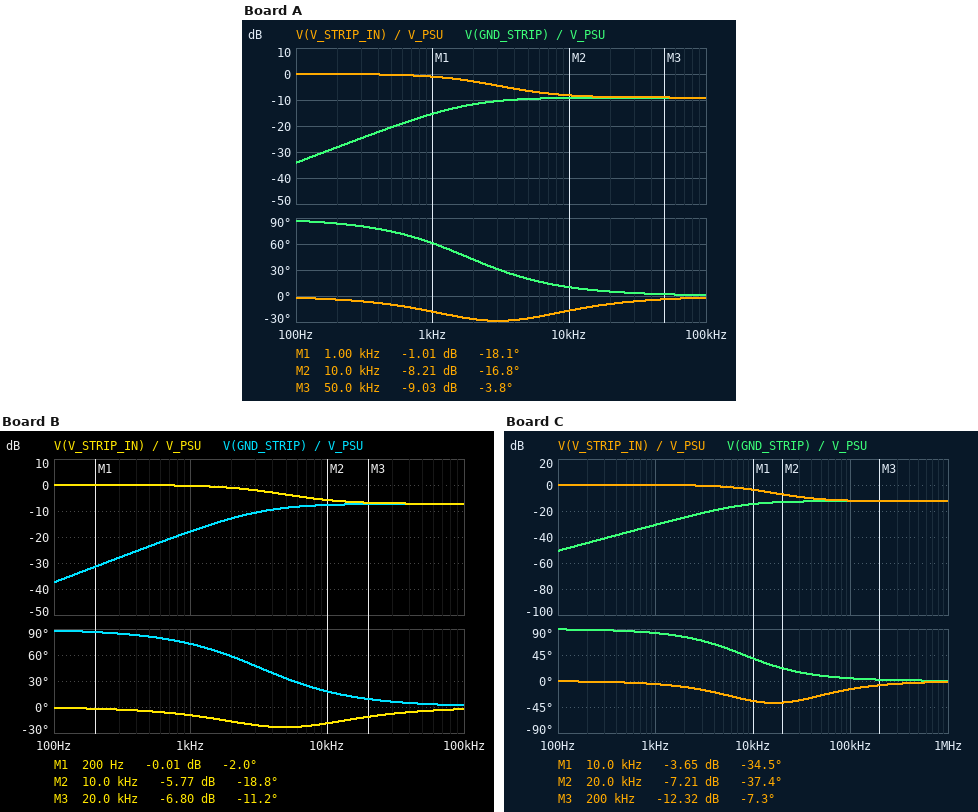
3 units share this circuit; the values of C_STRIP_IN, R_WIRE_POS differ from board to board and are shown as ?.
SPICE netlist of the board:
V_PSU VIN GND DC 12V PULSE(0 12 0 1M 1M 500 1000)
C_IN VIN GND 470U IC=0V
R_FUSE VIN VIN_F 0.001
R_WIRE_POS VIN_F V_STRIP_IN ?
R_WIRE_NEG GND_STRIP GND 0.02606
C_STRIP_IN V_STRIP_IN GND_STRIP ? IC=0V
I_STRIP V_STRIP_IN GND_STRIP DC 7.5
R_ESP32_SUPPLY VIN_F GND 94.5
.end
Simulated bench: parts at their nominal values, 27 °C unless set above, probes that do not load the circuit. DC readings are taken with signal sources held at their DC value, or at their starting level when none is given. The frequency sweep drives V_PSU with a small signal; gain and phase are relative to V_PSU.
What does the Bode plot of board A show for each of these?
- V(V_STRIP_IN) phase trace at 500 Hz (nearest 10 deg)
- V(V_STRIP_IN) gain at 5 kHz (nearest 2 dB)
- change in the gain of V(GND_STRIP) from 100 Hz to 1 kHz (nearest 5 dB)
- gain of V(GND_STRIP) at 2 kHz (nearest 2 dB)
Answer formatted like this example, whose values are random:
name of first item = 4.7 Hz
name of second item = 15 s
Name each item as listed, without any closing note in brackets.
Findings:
V(V_STRIP_IN) phase trace at 500 Hz = -10 deg
V(V_STRIP_IN) gain at 5 kHz = -6 dB
change in the gain of V(GND_STRIP) from 100 Hz to 1 kHz = 20 dB
gain of V(GND_STRIP) at 2 kHz = -12 dB
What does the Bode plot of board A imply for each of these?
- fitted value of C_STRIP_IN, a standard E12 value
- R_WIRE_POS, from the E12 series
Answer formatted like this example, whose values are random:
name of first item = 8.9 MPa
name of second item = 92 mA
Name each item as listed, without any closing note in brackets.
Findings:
fitted value of C_STRIP_IN, a standard E12 value = 1.2 mF
R_WIRE_POS, from the E12 series = 0.047 Ω
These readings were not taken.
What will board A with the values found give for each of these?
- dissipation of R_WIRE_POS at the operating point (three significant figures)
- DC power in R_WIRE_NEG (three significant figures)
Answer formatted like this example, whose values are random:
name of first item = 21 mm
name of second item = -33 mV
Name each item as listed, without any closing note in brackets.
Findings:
dissipation of R_WIRE_POS at the operating point = 2.64 W
DC power in R_WIRE_NEG = 1.47 W
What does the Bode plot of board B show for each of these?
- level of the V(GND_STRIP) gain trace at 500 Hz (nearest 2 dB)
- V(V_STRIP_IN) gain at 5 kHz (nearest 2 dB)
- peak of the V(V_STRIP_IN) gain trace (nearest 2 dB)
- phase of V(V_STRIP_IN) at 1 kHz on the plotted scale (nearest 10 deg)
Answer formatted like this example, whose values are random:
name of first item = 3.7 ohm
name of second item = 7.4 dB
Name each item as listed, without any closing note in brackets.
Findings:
level of the V(GND_STRIP) gain trace at 500 Hz = -24 dB
V(V_STRIP_IN) gain at 5 kHz = -4 dB
peak of the V(V_STRIP_IN) gain trace = 0 dB
phase of V(V_STRIP_IN) at 1 kHz on the plotted scale = -10 deg
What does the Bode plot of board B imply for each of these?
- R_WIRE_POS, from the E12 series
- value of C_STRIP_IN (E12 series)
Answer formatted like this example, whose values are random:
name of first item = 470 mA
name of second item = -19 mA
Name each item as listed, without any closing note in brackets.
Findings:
R_WIRE_POS, from the E12 series = 0.033 Ω
value of C_STRIP_IN = 820 µF
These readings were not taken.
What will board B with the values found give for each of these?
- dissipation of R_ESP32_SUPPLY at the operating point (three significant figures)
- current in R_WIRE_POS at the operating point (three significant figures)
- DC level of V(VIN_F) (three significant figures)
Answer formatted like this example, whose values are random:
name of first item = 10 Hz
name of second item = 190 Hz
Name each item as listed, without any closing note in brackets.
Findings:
dissipation of R_ESP32_SUPPLY at the operating point = 1.52 W
current in R_WIRE_POS at the operating point = 7.50 A
DC level of V(VIN_F) = 12.0 V
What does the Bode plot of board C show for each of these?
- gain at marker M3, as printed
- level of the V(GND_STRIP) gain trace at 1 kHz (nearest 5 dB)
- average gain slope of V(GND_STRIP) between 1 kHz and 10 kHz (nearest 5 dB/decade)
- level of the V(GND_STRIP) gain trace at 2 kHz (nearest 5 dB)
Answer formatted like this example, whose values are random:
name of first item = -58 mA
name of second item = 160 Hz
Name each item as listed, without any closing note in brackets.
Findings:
gain at marker M3, as printed = -12.32 dB
level of the V(GND_STRIP) gain trace at 1 kHz = -30 dB
average gain slope of V(GND_STRIP) between 1 kHz and 10 kHz = 15 dB/decade
level of the V(GND_STRIP) gain trace at 2 kHz = -25 dB
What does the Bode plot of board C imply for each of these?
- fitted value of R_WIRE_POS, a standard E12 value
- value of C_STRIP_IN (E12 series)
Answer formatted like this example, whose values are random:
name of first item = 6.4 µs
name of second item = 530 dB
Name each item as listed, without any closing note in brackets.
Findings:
fitted value of R_WIRE_POS, a standard E12 value = 0.082 Ω
value of C_STRIP_IN = 180 µF
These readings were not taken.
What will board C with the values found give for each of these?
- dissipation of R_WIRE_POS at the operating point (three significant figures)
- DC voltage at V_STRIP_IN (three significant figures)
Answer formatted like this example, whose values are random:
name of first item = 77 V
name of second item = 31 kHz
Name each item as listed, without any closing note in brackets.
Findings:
dissipation of R_WIRE_POS at the operating point = 4.61 W
DC voltage at V_STRIP_IN = 11.4 V
